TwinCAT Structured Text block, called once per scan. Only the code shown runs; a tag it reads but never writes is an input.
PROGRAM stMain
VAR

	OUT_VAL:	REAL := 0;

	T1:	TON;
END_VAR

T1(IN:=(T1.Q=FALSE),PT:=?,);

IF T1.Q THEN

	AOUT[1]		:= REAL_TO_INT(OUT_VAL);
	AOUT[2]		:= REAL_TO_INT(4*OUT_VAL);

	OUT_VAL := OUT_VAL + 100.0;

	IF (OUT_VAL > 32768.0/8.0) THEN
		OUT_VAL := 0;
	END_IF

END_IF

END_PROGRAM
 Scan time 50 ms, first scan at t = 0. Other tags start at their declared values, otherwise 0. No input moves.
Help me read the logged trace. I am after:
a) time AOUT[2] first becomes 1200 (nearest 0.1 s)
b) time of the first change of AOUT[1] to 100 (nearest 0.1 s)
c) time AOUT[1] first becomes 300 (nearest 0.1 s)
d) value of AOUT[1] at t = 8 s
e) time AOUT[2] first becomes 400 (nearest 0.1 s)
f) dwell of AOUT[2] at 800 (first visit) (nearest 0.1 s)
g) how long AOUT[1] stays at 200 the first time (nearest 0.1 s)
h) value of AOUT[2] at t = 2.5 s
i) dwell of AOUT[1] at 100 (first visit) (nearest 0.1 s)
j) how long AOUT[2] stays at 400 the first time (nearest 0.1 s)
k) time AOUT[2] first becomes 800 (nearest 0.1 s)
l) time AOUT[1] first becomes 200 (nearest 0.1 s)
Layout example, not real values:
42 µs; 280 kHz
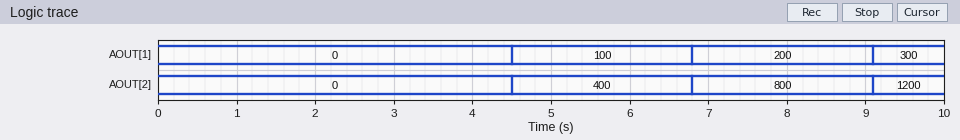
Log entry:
9.1 s; 4.5 s; 9.1 s; 200; 4.5 s; 2.3 s; 2.3 s; 0; 2.3 s; 2.3 s; 6.8 s; 6.8 s
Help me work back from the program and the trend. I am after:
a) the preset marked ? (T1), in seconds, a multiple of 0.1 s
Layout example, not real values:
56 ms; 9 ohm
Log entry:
2.2 s
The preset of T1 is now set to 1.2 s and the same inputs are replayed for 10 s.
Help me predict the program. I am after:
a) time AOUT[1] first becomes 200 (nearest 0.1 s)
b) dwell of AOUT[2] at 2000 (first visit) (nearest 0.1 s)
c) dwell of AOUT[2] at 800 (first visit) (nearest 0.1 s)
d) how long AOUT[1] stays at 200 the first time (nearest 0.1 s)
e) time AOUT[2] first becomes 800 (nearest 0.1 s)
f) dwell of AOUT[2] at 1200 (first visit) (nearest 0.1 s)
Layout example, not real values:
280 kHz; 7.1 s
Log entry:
3.8 s; 1.3 s; 1.3 s; 1.3 s; 3.8 s; 1.3 s
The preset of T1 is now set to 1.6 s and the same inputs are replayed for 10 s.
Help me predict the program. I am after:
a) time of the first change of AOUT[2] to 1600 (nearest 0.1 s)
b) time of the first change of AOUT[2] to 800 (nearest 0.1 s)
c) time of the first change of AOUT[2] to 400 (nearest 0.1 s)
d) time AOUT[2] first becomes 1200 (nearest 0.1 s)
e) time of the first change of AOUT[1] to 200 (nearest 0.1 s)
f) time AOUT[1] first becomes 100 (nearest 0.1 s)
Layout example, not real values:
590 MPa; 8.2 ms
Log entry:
8.4 s; 5.0 s; 3.3 s; 6.7 s; 5.0 s; 3.3 s
